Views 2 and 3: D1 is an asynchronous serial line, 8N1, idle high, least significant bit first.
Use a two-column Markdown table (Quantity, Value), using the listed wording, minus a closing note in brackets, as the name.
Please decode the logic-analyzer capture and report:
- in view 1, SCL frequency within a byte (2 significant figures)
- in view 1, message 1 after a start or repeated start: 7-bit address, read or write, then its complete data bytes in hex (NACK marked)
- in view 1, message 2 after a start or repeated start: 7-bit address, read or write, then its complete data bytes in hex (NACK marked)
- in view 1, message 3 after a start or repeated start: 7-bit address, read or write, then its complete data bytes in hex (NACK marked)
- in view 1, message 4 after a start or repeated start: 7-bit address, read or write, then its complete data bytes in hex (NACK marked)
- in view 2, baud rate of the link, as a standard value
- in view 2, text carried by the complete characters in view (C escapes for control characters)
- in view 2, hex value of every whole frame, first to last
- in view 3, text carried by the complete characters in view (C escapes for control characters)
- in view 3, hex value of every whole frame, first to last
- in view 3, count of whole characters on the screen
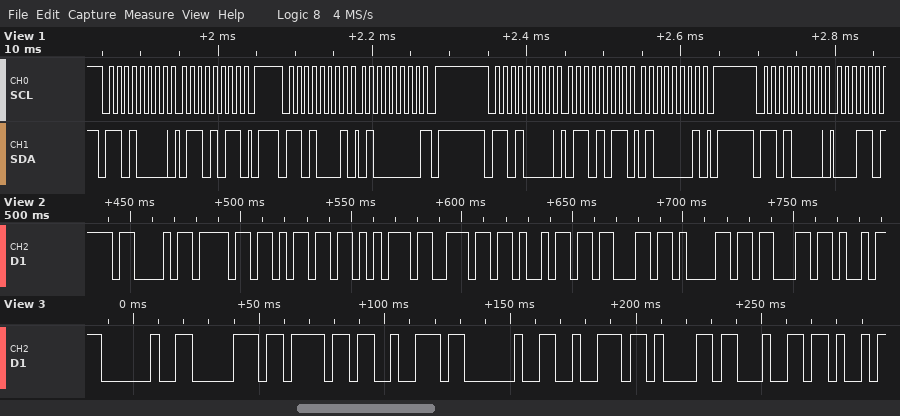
| Quantity | Value |
|---|---|
| in view 1, SCL frequency within a byte | 100 kHz |
| in view 1, message 1 after a start or repeated start: 7-bit address, read or write, then its complete data bytes in hex | 0x68 write: 6B |
| in view 1, message 2 after a start or repeated start: 7-bit address, read or write, then its complete data bytes in hex | 0x68 read: 40 NACK |
| in view 1, message 3 after a start or repeated start: 7-bit address, read or write, then its complete data bytes in hex | 0x68 write: 6B 41 |
| in view 1, message 4 after a start or repeated start: 7-bit address, read or write, then its complete data bytes in hex | 0x68 write |
| in view 2, baud rate of the link, as a standard value | 300 baud |
| in view 2, text carried by the complete characters in view | "Comunicac" |
| in view 2, hex value of every whole frame, first to last | 43 6F 6D 75 6E 69 63 61 63 |
| in view 3, text carried by the complete characters in view | " por rad" |
| in view 3, hex value of every whole frame, first to last | 0x20 0x70 0x6F 0x72 0x20 0x72 0x61 0x64 |
| in view 3, count of whole characters on the screen | 8 |
